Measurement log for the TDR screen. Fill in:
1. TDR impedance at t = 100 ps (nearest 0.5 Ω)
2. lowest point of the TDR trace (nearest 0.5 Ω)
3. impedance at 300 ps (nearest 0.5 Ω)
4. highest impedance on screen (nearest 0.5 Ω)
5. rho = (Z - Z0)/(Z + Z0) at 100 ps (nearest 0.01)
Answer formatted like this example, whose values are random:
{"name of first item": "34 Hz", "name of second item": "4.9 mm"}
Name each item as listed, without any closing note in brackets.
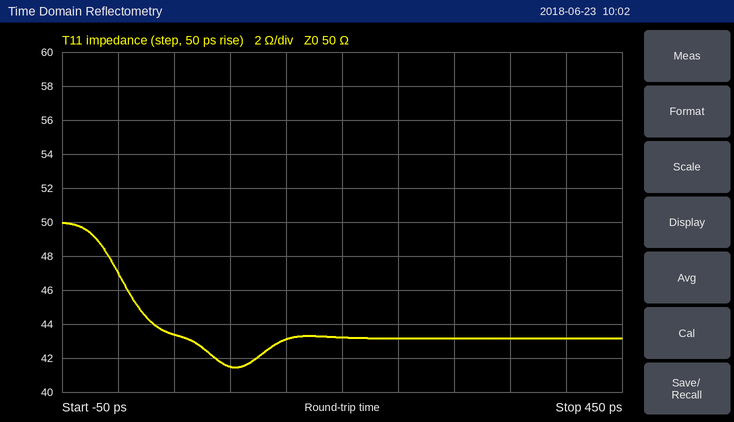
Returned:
{"TDR impedance at t = 100 ps": "41.5 Ω", "lowest point of the TDR trace": "41.5 Ω", "impedance at 300 ps": "43.0 Ω", "highest impedance on screen": "50.0 Ω", "rho = (Z - Z0)/(Z + Z0) at 100 ps": "-0.09"}
